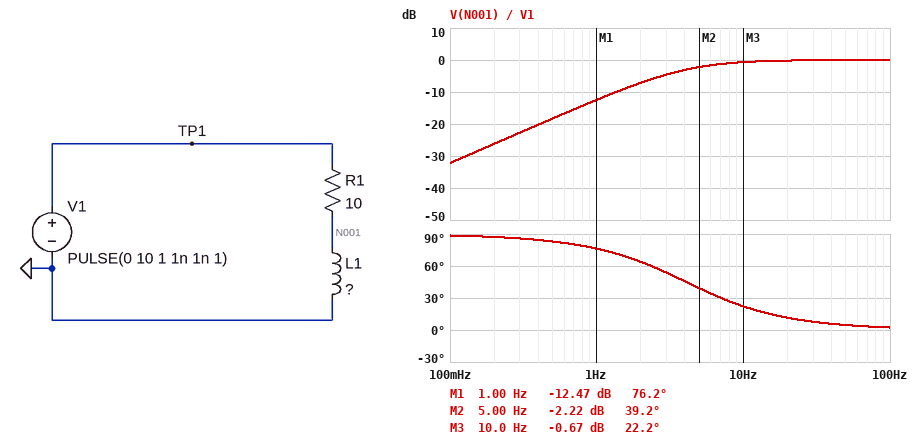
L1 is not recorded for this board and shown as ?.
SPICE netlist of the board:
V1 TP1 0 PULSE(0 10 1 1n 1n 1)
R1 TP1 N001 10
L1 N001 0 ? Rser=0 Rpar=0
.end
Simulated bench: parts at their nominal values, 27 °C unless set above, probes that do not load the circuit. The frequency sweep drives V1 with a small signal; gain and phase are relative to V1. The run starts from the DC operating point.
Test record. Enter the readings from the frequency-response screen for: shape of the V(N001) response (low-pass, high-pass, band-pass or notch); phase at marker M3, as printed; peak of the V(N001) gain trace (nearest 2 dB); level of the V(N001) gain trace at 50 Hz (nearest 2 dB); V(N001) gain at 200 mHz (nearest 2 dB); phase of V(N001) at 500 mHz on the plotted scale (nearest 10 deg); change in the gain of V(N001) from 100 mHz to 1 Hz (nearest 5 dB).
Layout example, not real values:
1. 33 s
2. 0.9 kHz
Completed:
1. high-pass
2. 22.2 deg
3. 0 dB
4. 0 dB
5. -26 dB
6. 80 deg
7. 20 dB
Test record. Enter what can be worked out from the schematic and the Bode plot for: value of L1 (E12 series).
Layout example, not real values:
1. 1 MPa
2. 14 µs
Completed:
1. 390 mH
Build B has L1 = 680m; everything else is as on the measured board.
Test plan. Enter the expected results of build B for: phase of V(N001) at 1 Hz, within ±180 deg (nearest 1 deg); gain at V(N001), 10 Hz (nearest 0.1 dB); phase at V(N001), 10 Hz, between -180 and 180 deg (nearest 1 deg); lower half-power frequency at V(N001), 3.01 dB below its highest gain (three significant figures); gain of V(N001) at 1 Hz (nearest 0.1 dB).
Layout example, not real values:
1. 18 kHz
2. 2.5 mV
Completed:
1. 67 deg
2. -0.2 dB
3. 13 deg
4. 2.34 Hz
5. -8.1 dB
